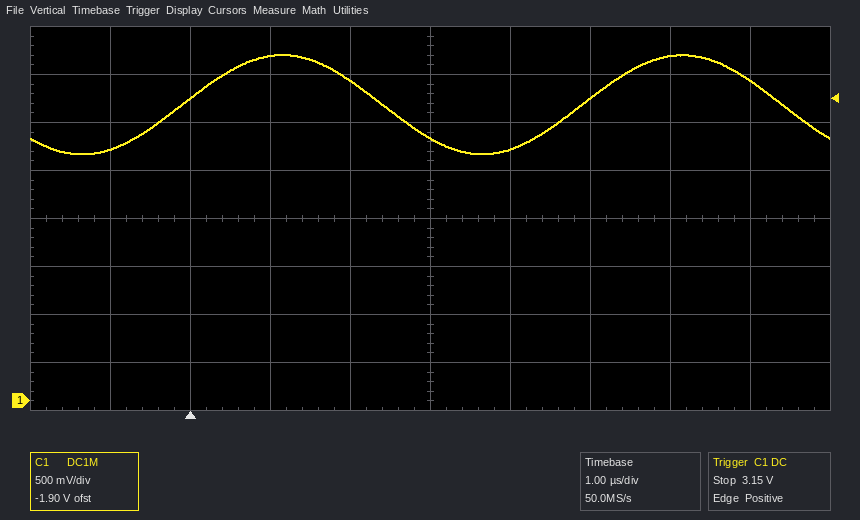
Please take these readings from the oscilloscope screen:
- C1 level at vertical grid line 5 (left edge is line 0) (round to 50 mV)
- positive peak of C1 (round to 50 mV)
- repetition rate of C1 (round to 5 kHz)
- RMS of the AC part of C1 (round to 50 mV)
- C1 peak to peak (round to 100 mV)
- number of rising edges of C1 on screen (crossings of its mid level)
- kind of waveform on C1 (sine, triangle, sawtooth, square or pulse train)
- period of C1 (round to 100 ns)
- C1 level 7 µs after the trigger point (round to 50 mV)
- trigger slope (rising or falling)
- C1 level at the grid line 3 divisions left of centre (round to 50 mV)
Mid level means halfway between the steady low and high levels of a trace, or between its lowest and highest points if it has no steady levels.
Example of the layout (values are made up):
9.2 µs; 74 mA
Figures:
2.75 V; 3.60 V; 200 kHz; 350 mV; 1.00 V; 2; sine; 5.0 µs; 3.35 V; rising; 3.15 V
